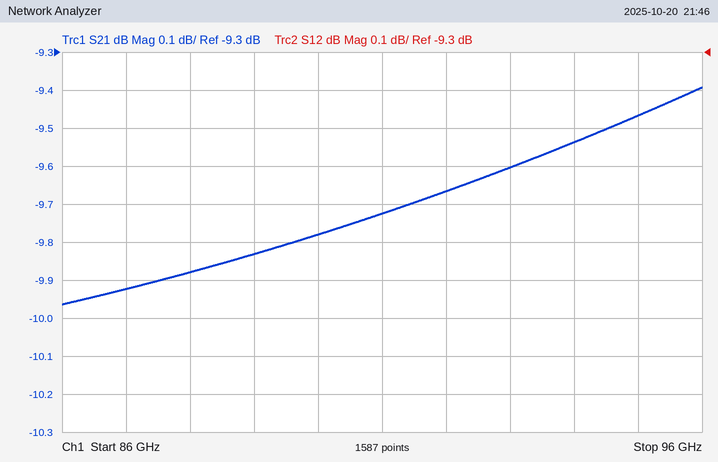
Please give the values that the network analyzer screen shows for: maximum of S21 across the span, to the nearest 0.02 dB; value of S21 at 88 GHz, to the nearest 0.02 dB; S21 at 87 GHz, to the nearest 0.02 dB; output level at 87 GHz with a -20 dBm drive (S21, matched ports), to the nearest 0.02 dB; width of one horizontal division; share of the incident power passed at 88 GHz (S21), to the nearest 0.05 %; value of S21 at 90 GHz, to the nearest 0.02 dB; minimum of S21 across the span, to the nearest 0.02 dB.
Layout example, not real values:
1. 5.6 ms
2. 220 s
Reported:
1. -9.40 dB
2. -9.88 dB
3. -9.92 dB
4. -29.92 dBm
5. 1 GHz
6. 10.30 %
7. -9.78 dB
8. -9.96 dB
